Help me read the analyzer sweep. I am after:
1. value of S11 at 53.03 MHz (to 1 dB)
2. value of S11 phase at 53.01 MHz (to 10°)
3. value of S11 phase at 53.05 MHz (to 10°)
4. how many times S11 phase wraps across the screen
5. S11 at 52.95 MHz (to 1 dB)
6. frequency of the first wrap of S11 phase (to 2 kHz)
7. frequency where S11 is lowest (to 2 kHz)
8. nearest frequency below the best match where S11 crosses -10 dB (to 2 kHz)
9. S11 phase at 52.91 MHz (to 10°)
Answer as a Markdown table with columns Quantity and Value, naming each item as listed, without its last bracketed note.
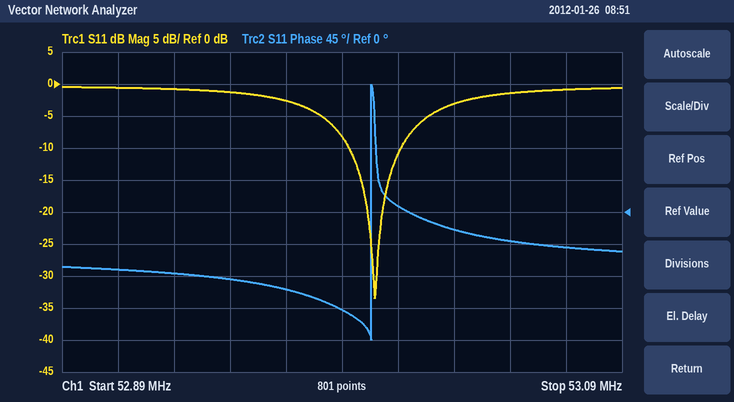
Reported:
| Quantity | Value |
|---|---|
| value of S11 at 53.03 MHz | -3 dB |
| value of S11 phase at 53.01 MHz | 10° |
| value of S11 phase at 53.05 MHz | -40° |
| how many times S11 phase wraps across the screen | 1 |
| S11 at 52.95 MHz | -1 dB |
| frequency of the first wrap of S11 phase | 53.000 MHz |
| frequency where S11 is lowest | 53.002 MHz |
| nearest frequency below the best match where S11 crosses -10 dB | 52.992 MHz |
| S11 phase at 52.91 MHz | -80° |
